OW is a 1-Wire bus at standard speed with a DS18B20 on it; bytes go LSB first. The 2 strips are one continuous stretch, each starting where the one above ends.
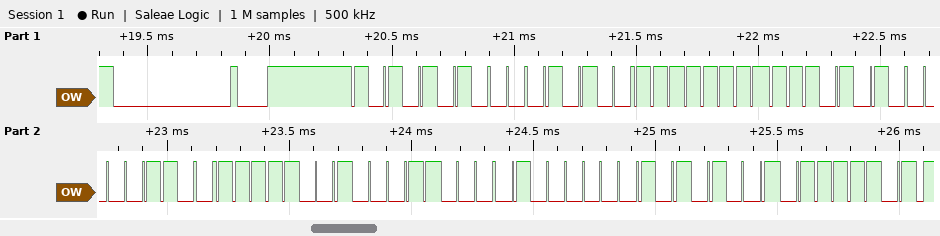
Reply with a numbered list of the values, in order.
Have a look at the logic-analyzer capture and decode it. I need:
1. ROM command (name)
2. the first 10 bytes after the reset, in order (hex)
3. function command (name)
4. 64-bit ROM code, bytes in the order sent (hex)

1. Match ROM
2. 55 28 FF 57 30 9F 18 02 95 BE
3. Read Scratchpad
4. 28 FF 57 30 9F 18 02 95
